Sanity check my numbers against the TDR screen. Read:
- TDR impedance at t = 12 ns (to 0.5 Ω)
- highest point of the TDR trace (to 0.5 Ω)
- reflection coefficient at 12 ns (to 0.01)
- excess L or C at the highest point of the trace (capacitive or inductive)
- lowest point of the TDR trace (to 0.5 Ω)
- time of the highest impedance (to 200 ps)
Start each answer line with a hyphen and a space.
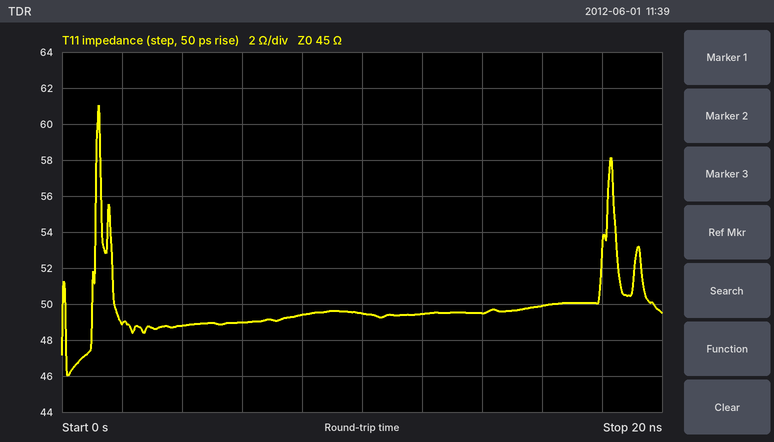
- 49.5 Ω
- 61.0 Ω
- +0.05
- inductive
- 46.0 Ω
- 1.2 ns
